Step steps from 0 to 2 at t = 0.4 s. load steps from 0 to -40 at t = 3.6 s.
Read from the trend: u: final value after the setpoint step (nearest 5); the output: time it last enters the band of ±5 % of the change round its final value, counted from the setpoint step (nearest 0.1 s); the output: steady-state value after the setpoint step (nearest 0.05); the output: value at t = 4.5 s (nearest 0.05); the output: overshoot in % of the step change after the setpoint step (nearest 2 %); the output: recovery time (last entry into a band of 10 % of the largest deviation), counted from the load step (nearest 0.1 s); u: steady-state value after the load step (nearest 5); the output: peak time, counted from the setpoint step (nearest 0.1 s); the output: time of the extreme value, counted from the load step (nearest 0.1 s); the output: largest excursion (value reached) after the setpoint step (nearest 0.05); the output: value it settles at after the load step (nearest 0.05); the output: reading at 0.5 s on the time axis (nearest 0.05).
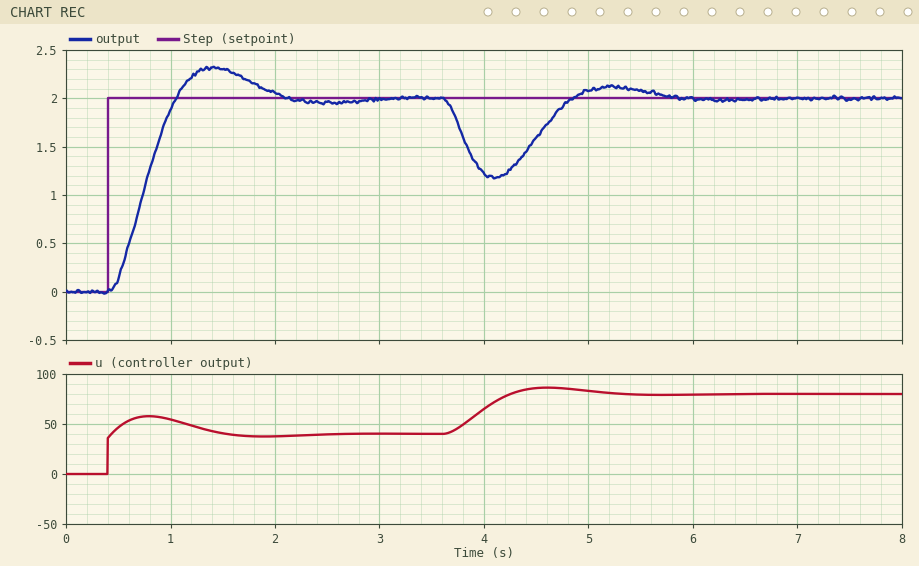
40
1.5 s
2.00
1.60
16 %
1.9 s
80
1.0 s
0.5 s
2.30
2.00
0.15
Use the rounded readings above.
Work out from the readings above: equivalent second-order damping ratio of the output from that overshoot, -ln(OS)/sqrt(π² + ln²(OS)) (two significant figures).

0.50
